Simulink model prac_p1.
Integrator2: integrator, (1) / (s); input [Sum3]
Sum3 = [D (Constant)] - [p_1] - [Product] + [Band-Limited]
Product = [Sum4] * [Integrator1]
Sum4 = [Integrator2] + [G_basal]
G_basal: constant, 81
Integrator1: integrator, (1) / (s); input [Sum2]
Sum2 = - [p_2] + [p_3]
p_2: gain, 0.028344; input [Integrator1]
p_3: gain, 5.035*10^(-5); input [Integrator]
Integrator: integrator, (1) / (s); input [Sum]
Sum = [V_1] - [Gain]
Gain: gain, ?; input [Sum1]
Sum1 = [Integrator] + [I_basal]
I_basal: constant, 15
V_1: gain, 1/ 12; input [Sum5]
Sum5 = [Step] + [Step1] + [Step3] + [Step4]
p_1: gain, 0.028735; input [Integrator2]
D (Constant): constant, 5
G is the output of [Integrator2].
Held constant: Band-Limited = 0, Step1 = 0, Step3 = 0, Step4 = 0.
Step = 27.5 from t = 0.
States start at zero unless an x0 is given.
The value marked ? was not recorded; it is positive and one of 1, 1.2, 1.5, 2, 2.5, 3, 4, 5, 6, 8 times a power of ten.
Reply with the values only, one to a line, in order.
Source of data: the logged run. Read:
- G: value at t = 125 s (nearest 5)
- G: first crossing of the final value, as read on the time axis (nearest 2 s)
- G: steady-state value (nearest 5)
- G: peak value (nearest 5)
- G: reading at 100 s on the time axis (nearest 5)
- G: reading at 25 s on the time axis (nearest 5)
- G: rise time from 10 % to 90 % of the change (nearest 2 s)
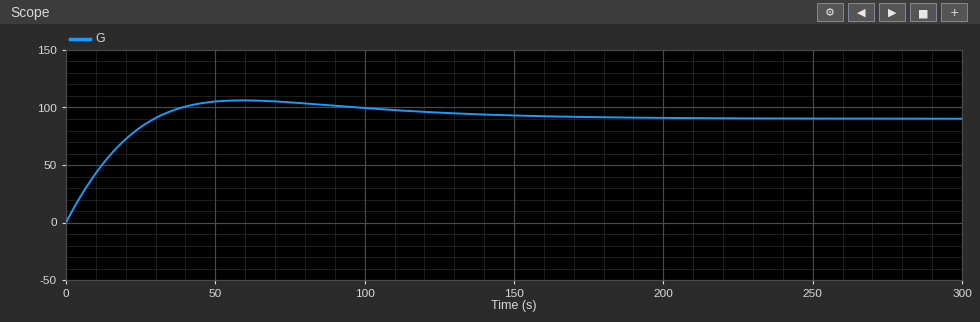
95
30 s
90
105
100
85
22 s
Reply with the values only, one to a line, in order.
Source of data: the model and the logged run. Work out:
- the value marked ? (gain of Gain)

0.1
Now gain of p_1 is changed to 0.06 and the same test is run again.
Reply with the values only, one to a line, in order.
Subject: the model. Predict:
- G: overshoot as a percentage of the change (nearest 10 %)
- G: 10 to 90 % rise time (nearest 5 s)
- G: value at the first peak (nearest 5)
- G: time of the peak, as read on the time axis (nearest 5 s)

20 %
15 s
65
40 s
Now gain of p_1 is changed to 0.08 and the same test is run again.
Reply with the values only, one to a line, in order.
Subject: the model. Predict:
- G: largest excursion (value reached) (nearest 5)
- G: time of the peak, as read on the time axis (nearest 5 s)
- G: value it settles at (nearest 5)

50
35 s
40
